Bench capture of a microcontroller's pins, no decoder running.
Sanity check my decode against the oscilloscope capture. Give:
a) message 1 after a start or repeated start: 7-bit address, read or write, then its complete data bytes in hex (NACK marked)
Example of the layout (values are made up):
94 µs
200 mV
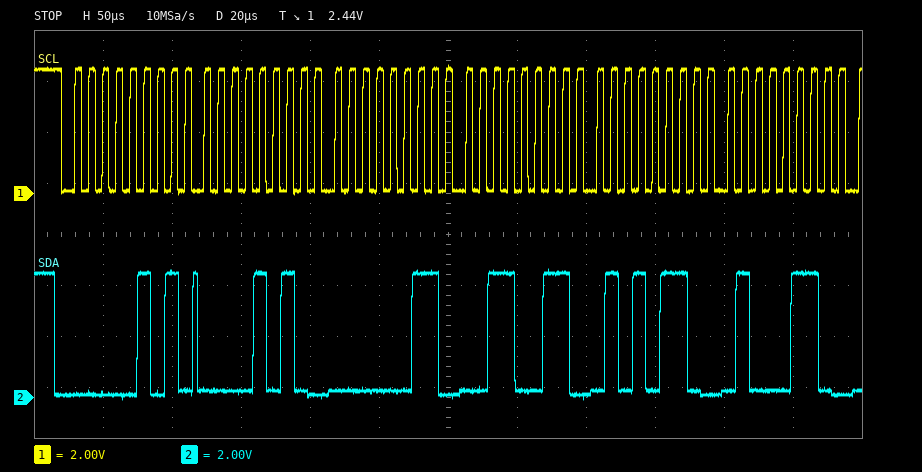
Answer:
0x02 read: 0A 03 33 56 46
